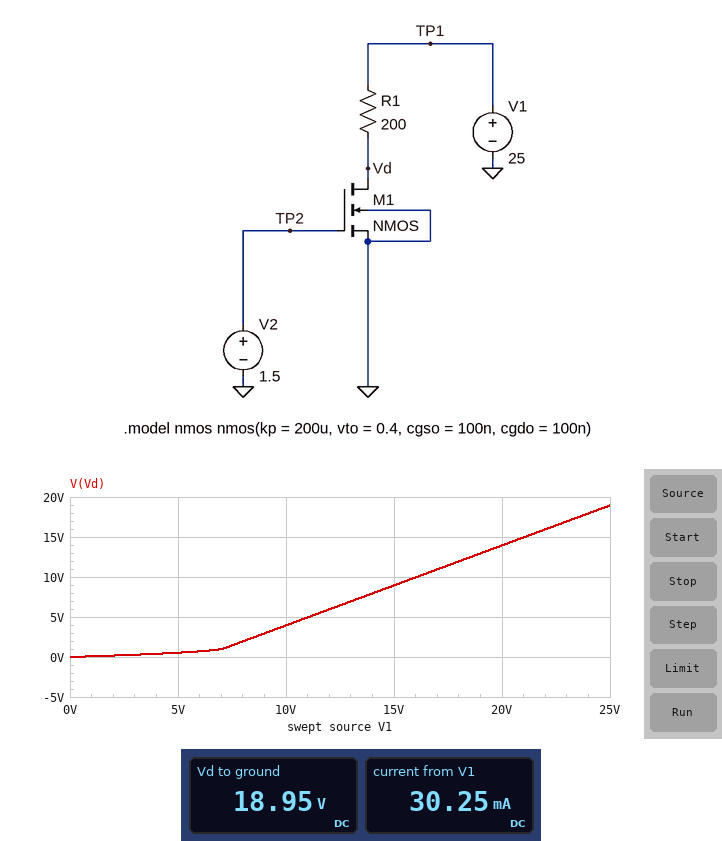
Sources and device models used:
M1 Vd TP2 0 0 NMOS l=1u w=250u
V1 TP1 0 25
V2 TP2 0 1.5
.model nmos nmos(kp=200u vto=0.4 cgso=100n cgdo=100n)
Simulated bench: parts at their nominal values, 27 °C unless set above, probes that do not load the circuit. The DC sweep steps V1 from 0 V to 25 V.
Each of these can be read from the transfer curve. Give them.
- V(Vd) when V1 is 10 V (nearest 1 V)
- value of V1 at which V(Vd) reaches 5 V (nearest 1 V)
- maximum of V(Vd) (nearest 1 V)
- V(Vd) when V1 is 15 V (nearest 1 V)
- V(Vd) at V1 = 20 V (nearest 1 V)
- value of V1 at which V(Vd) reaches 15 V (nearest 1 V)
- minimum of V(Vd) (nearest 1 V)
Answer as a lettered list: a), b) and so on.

a) 4 V
b) 11 V
c) 19 V
d) 9 V
e) 14 V
f) 21 V
g) 0 V
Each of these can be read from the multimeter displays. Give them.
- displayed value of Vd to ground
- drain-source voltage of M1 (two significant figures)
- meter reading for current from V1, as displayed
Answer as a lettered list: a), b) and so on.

a) 18.95 V
b) 19 V
c) 30.25 mA
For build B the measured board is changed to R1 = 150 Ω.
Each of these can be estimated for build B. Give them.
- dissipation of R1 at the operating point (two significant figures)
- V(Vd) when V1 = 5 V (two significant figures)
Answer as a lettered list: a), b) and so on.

a) 140 mW
b) 800 mV
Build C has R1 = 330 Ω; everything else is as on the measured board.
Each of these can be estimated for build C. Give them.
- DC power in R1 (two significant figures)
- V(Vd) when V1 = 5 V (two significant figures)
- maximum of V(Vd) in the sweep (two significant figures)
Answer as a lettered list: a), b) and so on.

a) 300 mW
b) 300 mV
c) 15 V
